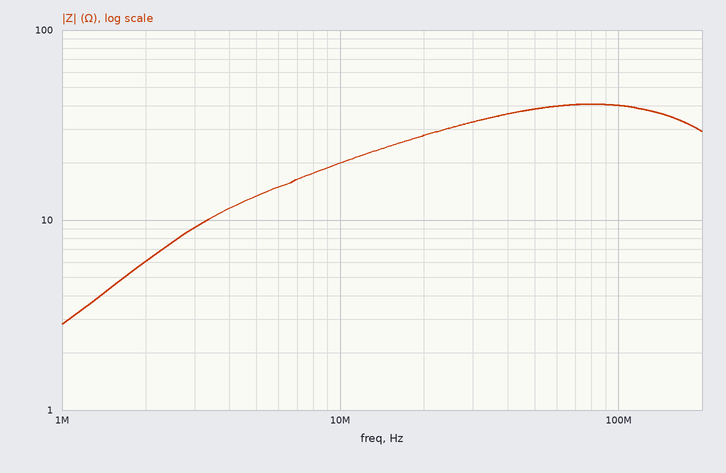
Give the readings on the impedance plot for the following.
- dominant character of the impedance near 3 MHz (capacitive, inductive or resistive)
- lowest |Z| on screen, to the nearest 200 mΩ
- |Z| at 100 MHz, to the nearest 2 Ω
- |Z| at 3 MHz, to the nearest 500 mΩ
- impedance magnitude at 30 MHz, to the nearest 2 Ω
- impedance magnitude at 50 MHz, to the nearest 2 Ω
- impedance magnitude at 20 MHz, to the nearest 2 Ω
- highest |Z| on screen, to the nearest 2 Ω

inductive
2.8 Ω
40 Ω
9.0 Ω
32 Ω
38 Ω
28 Ω
40 Ω
